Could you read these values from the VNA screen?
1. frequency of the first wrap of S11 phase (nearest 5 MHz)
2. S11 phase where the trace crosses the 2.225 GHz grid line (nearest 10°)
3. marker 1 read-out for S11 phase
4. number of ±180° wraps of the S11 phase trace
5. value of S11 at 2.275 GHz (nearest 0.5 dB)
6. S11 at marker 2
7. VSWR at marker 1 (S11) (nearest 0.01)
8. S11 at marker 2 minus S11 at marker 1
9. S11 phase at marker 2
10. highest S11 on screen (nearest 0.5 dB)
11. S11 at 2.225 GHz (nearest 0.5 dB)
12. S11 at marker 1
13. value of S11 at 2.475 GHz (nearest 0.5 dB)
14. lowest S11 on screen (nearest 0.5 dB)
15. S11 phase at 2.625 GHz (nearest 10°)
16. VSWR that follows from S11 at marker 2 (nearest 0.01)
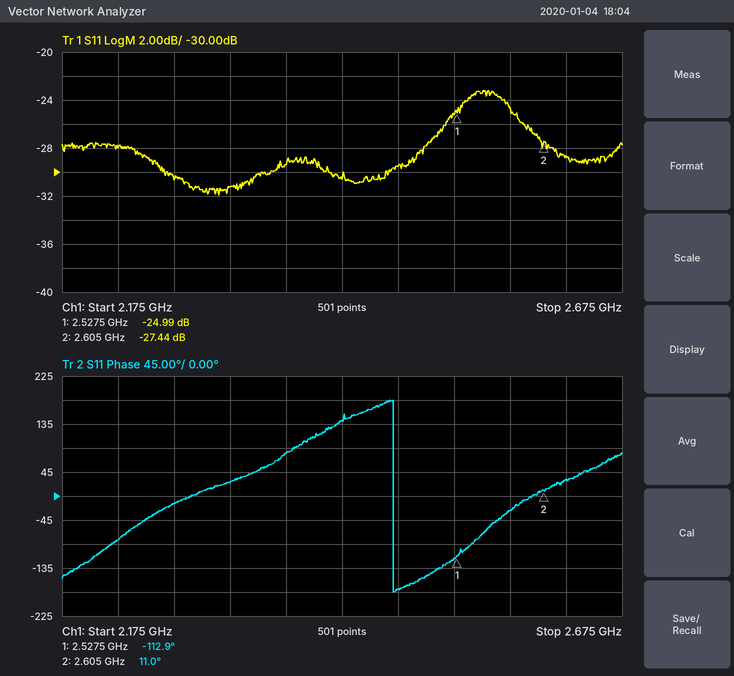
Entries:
2.470 GHz
-80°
-112.9°
1
-30.5 dB
-27.44 dB
1.12
-2.45 dB
11.0°
-23.0 dB
-28.0 dB
-24.99 dB
-29.5 dB
-32.0 dB
30°
1.09
